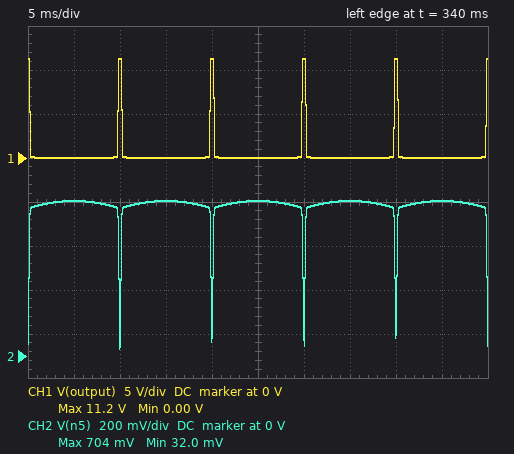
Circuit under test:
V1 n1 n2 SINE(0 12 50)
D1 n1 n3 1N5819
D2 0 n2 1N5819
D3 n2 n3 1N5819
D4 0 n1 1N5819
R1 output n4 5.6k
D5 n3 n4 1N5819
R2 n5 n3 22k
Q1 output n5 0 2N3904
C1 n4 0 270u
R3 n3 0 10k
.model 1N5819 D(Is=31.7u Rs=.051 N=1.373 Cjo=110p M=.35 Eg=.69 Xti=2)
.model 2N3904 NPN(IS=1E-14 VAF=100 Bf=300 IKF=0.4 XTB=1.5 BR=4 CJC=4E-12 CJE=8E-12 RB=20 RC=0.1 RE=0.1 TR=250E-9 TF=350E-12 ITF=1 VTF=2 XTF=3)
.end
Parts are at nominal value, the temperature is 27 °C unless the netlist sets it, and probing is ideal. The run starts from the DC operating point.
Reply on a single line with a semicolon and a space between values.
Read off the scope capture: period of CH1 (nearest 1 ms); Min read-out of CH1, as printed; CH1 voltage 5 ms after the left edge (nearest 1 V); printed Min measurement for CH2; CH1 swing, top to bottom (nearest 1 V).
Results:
10 ms; 0.00 V; 0 V; 32.0 mV; 11 V
